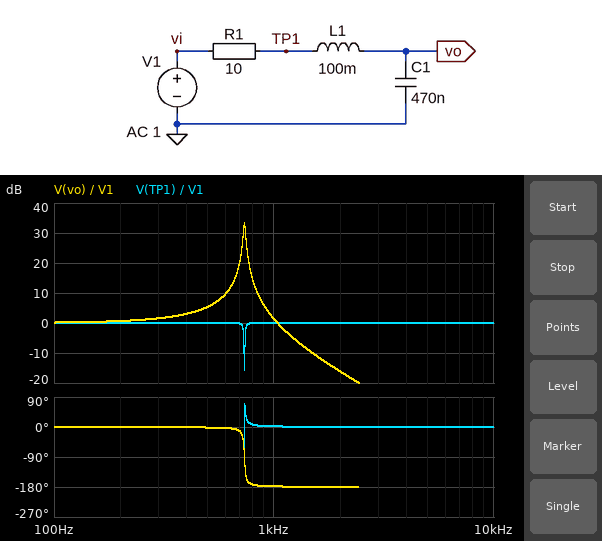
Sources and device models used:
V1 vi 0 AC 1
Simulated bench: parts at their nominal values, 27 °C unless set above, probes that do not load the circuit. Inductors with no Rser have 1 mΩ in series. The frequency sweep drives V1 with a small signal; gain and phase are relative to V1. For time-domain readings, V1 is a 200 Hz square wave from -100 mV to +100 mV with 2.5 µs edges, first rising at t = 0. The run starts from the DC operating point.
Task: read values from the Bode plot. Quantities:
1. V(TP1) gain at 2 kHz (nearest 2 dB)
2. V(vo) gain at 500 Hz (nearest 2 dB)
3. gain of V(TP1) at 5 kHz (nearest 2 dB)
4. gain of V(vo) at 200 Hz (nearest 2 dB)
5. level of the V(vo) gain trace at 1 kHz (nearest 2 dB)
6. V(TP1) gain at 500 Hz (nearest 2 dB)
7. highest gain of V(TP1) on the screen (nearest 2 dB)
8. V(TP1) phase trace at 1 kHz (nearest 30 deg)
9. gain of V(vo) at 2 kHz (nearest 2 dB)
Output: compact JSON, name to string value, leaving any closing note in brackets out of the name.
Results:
{"V(TP1) gain at 2 kHz": "0 dB", "V(vo) gain at 500 Hz": "6 dB", "gain of V(TP1) at 5 kHz": "0 dB", "gain of V(vo) at 200 Hz": "0 dB", "level of the V(vo) gain trace at 1 kHz": "2 dB", "V(TP1) gain at 500 Hz": "0 dB", "highest gain of V(TP1) on the screen": "0 dB", "V(TP1) phase trace at 1 kHz": "0 deg", "gain of V(vo) at 2 kHz": "-16 dB"}
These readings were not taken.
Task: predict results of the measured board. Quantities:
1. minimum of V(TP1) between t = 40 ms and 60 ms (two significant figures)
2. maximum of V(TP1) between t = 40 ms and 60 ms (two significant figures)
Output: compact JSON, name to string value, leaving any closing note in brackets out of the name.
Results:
{"minimum of V(TP1) between t = 40 ms and 60 ms": "-100 mV", "maximum of V(TP1) between t = 40 ms and 60 ms": "100 mV"}
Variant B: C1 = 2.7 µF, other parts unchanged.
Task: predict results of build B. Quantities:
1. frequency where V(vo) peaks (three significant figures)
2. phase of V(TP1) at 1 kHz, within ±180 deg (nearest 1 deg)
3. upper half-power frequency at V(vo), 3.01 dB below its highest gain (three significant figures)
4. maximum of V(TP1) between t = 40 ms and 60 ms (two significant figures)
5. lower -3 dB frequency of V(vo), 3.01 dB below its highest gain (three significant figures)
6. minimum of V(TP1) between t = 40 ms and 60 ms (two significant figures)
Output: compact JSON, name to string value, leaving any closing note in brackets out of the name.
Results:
{"frequency where V(vo) peaks": "306 Hz", "phase of V(TP1) at 1 kHz, within ±180 deg": "1 deg", "upper half-power frequency at V(vo), 3.01 dB below its highest gain": "314 Hz", "maximum of V(TP1) between t = 40 ms and 60 ms": "110 mV", "lower -3 dB frequency of V(vo), 3.01 dB below its highest gain": "298 Hz", "minimum of V(TP1) between t = 40 ms and 60 ms": "-110 mV"}
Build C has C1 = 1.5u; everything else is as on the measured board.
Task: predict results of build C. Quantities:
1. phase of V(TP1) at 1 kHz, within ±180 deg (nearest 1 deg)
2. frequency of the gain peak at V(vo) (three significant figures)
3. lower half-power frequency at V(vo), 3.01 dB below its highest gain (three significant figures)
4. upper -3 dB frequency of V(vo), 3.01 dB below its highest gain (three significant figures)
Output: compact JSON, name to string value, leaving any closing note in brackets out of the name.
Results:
{"phase of V(TP1) at 1 kHz, within ±180 deg": "1 deg", "frequency of the gain peak at V(vo)": "411 Hz", "lower half-power frequency at V(vo), 3.01 dB below its highest gain": "403 Hz", "upper -3 dB frequency of V(vo), 3.01 dB below its highest gain": "419 Hz"}
